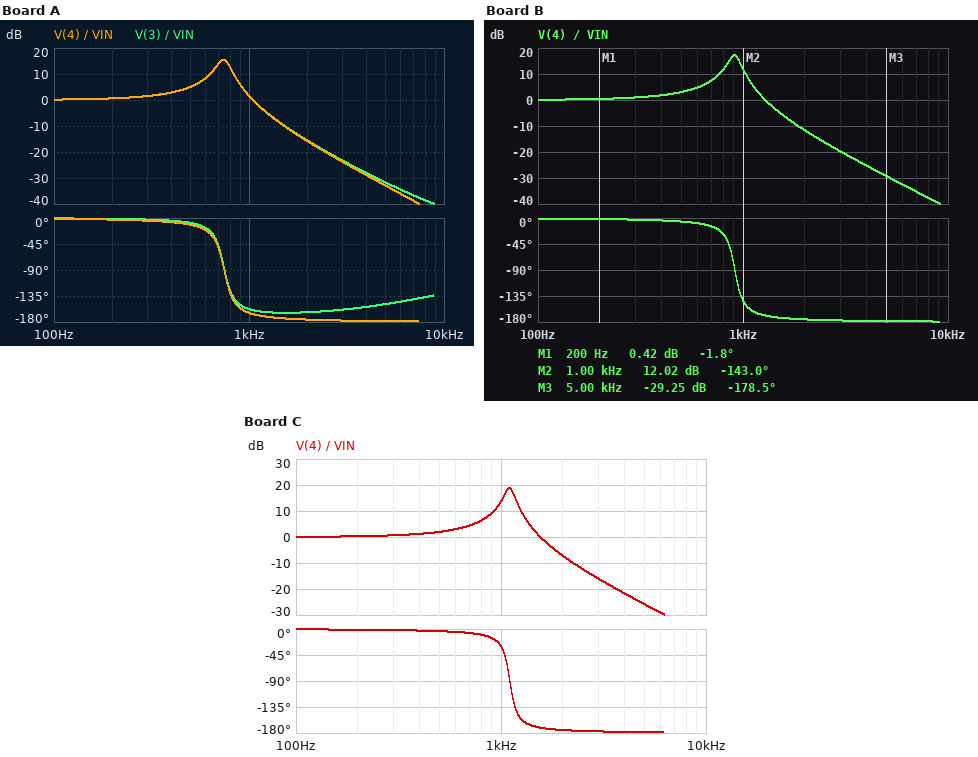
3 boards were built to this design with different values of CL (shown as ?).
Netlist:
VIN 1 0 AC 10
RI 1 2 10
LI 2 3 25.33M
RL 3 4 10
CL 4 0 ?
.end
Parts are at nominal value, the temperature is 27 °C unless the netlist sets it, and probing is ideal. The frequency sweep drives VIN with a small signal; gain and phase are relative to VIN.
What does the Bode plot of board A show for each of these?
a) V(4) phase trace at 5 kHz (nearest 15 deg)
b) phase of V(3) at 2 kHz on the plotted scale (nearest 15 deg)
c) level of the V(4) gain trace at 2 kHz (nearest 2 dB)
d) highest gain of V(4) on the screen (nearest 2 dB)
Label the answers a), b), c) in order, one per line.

a) -180 deg
b) -165 deg
c) -16 dB
d) 16 dB
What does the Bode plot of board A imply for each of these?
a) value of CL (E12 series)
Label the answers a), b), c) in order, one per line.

a) 1.8 µF
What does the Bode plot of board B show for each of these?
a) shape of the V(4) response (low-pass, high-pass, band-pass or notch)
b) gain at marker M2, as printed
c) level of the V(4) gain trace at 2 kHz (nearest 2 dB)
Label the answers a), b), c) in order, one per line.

a) low-pass
b) 12.02 dB
c) -12 dB
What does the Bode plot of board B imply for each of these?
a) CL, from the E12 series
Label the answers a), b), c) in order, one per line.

a) 1.2 µF
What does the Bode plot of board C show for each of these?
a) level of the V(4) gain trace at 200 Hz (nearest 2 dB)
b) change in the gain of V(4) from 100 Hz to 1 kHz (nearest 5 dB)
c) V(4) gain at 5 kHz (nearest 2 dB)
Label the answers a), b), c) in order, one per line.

a) 0 dB
b) 15 dB
c) -26 dB
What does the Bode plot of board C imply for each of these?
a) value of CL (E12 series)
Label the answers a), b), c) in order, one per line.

a) 820 nF
